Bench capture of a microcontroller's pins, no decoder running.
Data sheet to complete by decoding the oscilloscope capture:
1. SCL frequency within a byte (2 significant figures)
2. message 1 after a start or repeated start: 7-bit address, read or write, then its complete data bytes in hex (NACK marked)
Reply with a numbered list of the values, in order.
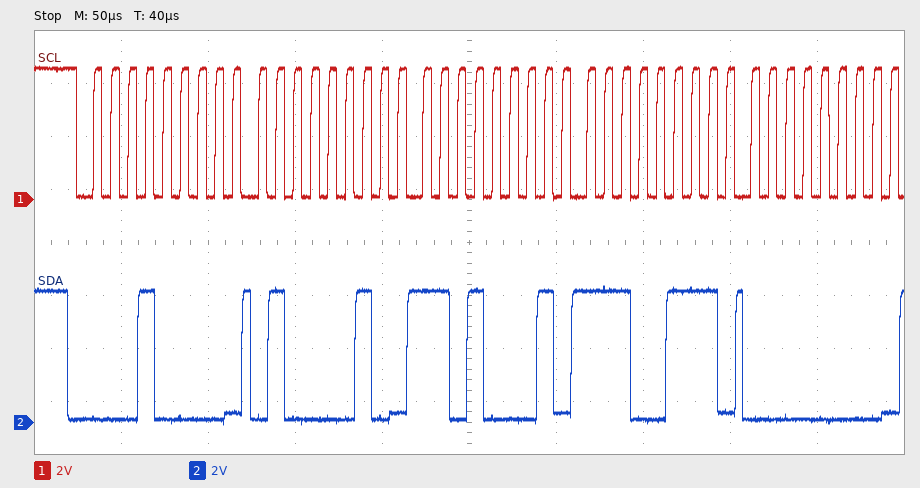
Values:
1. 100 kHz
2. 0x08 write: 42 D1 E7 00
